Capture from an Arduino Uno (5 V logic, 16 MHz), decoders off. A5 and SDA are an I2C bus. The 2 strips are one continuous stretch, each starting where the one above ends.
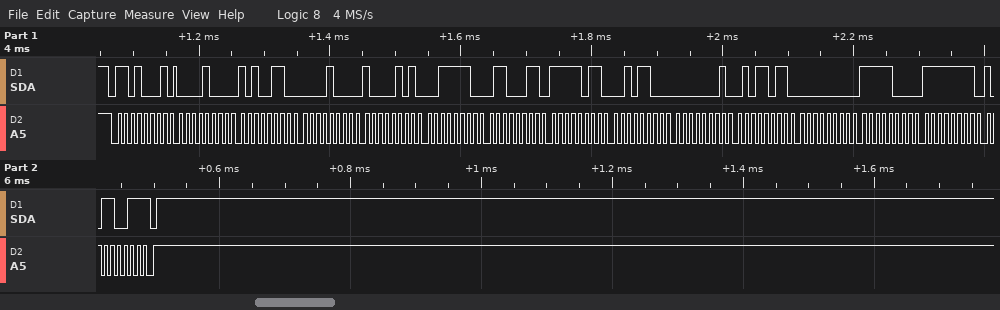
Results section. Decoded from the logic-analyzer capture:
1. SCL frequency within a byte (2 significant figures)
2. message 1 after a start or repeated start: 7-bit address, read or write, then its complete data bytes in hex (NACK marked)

100 kHz
0x68 read: 08 A6 08 85 3E 63 FB 2C 01 5B 00 F8 FF B3 NACK
